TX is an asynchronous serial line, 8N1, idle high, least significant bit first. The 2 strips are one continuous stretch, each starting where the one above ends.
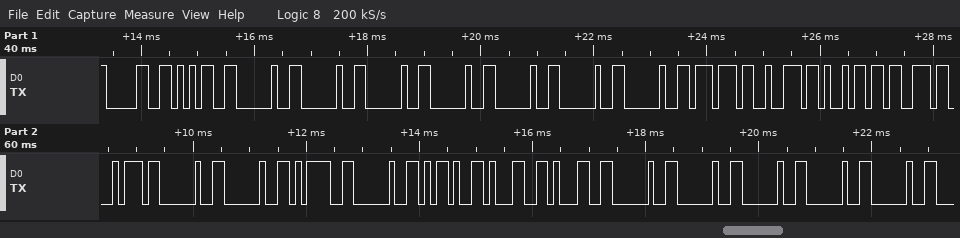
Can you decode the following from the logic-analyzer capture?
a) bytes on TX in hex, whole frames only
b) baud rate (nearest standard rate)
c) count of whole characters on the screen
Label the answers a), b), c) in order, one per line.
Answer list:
a) 30 35 20 20 20 20 20 20 20 77 72 69 73 74 20 20 3D 20 2D 31 31 20 20 20 20 20
b) 9600 baud
c) 26
